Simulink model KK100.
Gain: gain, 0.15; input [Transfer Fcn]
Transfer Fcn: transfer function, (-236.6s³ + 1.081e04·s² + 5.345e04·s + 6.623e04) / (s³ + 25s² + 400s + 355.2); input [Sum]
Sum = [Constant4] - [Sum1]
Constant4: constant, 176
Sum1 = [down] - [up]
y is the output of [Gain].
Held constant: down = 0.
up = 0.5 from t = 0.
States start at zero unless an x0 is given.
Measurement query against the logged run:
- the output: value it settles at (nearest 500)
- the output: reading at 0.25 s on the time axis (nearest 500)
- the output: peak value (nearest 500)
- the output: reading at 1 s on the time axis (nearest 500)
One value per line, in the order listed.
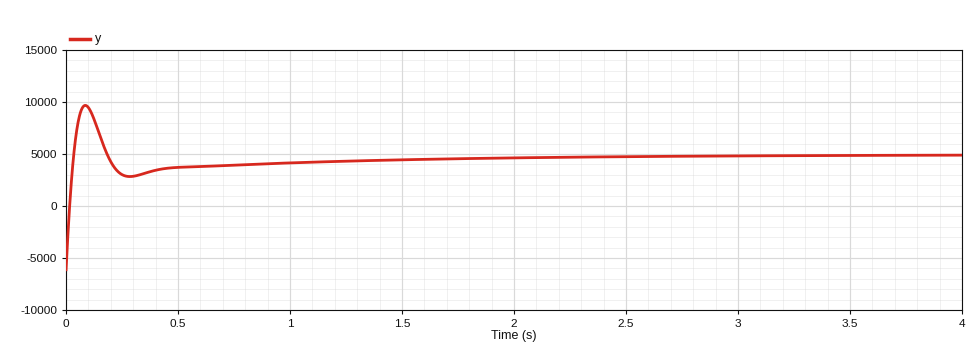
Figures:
5000
3000
9500
4000
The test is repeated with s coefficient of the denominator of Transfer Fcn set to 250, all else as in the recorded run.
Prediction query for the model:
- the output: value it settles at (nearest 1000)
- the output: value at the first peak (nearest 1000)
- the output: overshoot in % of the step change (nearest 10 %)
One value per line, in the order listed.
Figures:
5000
11000
50 %
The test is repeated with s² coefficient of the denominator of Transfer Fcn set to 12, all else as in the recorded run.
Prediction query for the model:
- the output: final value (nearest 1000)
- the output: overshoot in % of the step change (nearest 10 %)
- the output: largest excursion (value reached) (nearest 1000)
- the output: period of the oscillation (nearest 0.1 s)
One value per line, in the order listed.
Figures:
5000
80 %
14000
0.3 s
